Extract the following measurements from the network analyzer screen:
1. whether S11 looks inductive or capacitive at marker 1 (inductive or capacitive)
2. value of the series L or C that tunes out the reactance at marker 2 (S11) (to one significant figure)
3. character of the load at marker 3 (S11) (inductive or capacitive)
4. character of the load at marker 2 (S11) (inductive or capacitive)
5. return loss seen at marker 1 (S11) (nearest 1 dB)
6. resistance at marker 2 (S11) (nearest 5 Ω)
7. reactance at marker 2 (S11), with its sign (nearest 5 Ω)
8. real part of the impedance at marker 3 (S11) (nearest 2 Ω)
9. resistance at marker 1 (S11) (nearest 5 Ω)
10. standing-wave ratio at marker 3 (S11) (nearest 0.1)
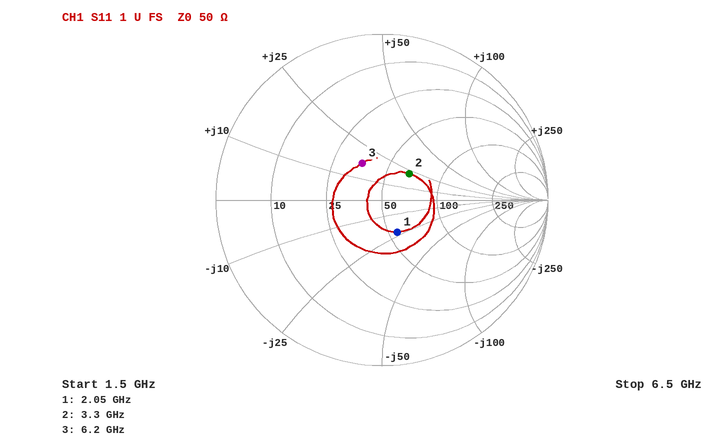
capacitive
2 pF
inductive
inductive
13 dB
65 Ω
+20 Ω
36 Ω
55 Ω
1.7
